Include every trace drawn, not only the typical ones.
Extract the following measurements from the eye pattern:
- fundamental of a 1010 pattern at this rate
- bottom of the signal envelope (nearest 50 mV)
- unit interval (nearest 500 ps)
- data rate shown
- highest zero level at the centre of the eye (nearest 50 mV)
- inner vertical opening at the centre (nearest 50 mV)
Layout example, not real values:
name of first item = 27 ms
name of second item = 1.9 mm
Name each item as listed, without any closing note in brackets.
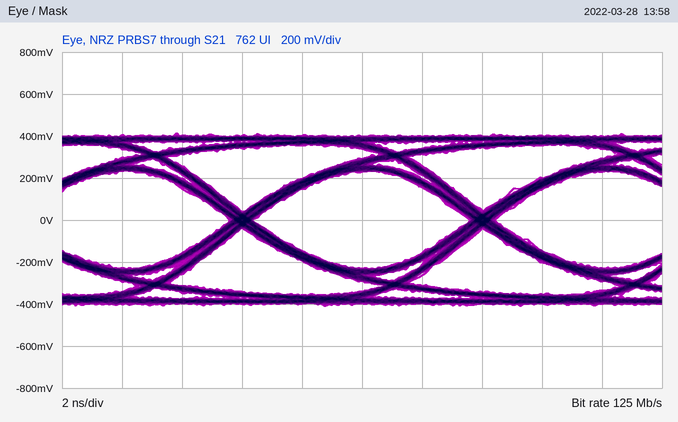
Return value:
fundamental of a 1010 pattern at this rate = 62.5 MHz
bottom of the signal envelope = -400 mV
unit interval = 8.0 ns
data rate shown = 125 Mb/s
highest zero level at the centre of the eye = -250 mV
inner vertical opening at the centre = 450 mV
